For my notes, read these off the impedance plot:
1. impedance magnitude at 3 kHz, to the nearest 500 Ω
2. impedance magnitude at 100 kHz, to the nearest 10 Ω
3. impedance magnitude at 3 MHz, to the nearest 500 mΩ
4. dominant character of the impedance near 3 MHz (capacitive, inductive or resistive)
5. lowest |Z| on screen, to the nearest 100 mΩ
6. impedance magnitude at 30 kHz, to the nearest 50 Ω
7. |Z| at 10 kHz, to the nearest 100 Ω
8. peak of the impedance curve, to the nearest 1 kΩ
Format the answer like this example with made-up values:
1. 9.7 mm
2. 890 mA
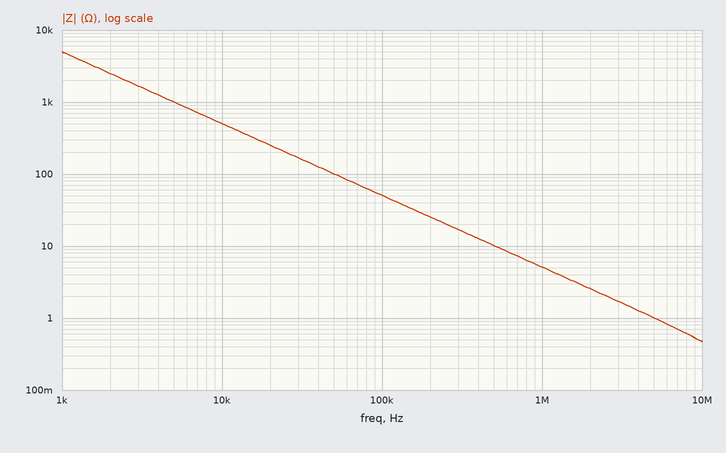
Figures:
1. 1.5 kΩ
2. 50 Ω
3. 1.5 Ω
4. capacitive
5. 500 mΩ
6. 150 Ω
7. 500 Ω
8. 5 kΩ
